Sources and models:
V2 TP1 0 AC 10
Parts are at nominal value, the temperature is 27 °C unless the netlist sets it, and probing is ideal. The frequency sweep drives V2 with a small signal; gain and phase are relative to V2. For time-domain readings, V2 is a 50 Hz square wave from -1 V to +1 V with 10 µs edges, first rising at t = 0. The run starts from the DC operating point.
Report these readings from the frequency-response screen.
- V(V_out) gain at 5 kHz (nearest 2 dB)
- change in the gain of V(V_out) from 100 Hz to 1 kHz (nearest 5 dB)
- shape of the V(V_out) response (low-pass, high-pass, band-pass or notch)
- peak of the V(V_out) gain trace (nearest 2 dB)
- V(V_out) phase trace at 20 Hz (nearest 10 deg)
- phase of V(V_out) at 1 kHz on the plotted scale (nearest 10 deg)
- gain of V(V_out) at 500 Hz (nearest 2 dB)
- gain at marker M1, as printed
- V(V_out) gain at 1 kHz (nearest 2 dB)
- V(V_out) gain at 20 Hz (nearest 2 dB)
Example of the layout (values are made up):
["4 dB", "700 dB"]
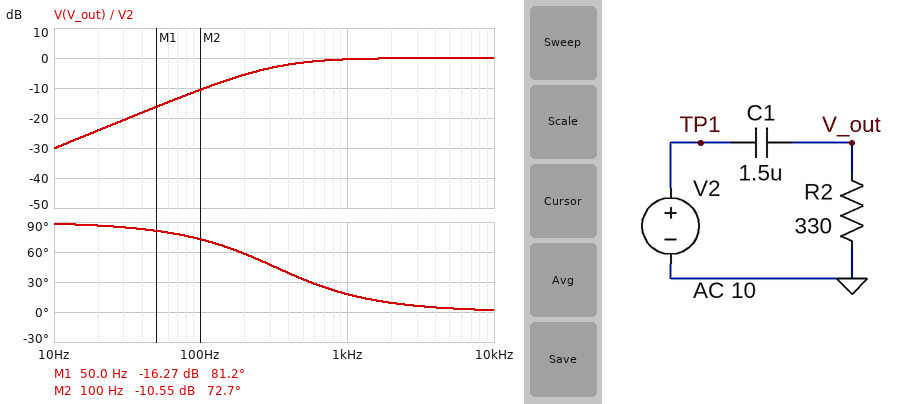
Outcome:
["0 dB", "10 dB", "high-pass", "0 dB", "90 deg", "20 deg", "-2 dB", "-16.27 dB", "0 dB", "-24 dB"]
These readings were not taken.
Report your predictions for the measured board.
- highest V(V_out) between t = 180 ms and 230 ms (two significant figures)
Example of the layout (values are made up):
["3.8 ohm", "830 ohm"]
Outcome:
["2.0 V"]
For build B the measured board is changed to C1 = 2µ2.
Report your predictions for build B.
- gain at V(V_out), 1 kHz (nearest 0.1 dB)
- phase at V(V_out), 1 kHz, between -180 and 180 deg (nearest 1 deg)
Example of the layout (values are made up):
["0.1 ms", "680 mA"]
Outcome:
["-0.2 dB", "12 deg"]
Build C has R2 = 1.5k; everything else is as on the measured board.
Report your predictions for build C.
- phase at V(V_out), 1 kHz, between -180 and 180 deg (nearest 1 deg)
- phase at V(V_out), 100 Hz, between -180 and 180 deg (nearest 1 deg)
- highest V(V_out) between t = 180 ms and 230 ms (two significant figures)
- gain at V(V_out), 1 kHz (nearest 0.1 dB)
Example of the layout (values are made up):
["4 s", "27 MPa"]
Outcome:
["4 deg", "35 deg", "2.0 V", "0 dB"]
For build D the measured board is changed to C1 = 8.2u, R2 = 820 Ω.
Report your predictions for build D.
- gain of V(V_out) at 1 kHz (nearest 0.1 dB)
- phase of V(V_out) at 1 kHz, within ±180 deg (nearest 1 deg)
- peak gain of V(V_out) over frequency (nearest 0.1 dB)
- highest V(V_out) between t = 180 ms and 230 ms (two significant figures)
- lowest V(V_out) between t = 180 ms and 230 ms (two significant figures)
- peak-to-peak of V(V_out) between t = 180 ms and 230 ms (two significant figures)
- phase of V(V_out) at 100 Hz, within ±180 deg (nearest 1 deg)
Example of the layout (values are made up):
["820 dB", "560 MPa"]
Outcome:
["0 dB", "1 deg", "0 dB", "1.6 V", "-1.6 V", "3.3 V", "13 deg"]
